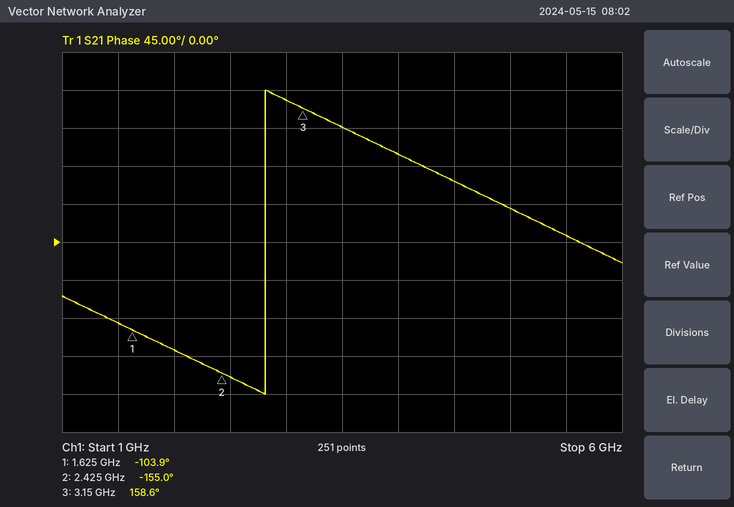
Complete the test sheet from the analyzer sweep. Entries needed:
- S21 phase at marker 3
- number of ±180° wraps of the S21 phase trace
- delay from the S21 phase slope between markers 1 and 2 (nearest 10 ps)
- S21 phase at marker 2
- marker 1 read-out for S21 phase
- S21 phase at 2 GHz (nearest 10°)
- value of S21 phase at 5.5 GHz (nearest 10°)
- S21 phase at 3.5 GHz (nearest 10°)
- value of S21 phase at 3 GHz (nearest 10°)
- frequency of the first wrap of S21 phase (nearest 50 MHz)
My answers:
158.6°
1
180 ps
-155.0°
-103.9°
-130°
10°
140°
170°
2.80 GHz
